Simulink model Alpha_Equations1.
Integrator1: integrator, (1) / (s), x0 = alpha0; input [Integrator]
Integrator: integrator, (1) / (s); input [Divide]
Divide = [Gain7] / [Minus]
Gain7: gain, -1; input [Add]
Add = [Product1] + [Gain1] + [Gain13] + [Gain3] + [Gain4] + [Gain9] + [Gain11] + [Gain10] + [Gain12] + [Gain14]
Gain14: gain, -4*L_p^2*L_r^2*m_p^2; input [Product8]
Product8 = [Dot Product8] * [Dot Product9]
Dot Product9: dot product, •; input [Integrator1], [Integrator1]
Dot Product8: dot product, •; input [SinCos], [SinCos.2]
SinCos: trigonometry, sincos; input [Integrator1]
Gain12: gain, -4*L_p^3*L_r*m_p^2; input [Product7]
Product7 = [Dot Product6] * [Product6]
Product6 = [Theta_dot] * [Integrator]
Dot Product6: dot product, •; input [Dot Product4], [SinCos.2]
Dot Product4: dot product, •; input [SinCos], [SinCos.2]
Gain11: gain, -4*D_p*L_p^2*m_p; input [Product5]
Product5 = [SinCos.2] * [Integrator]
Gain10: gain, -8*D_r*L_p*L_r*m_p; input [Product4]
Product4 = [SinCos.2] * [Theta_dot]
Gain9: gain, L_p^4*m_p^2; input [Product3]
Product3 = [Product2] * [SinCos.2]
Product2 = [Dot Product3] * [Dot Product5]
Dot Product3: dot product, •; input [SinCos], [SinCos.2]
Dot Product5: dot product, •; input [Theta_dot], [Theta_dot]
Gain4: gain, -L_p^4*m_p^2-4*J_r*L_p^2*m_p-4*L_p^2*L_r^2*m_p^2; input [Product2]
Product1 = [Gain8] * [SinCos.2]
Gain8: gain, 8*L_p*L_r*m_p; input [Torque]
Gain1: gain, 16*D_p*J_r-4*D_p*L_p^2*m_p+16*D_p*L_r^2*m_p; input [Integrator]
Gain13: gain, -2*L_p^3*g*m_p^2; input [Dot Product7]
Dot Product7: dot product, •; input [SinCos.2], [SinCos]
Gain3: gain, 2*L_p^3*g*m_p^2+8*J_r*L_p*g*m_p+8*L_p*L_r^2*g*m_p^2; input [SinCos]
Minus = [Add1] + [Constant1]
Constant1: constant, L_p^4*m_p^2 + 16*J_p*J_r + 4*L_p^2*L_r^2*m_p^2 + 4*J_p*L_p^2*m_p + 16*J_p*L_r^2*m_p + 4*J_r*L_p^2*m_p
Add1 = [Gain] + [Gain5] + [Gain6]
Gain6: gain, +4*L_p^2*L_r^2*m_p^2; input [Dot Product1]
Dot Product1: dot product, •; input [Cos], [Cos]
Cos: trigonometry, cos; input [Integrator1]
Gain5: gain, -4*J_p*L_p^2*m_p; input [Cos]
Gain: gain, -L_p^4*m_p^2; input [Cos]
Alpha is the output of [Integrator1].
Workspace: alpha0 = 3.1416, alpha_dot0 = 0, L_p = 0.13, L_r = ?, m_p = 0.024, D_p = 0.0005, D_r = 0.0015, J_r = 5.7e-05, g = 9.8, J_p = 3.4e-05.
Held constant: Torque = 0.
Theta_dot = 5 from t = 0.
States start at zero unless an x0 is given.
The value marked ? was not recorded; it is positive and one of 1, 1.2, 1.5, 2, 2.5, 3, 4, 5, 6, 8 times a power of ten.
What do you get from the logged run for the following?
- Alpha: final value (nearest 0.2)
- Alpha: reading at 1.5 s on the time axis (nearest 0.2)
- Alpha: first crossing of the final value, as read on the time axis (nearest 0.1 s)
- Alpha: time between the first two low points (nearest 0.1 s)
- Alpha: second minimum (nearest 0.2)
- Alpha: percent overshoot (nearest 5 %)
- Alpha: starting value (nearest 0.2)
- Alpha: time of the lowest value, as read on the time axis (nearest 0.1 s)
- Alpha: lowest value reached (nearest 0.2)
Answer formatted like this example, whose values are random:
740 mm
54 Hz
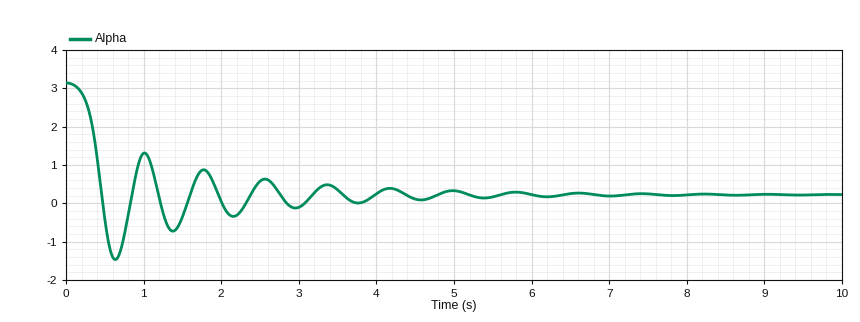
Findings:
0.2
-0.4
0.5 s
0.7 s
-0.8
60 %
3.2
0.6 s
-1.4
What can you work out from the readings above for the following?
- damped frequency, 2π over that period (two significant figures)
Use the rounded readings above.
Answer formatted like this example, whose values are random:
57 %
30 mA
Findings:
9.0 rad/s
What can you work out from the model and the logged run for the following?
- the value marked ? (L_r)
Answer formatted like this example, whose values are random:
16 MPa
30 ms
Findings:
0.15
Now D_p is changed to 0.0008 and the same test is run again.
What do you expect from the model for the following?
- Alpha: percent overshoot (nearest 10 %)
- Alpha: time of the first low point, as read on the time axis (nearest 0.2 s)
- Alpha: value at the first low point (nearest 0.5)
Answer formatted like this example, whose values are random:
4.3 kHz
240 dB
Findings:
50 %
0.6 s
-1.0
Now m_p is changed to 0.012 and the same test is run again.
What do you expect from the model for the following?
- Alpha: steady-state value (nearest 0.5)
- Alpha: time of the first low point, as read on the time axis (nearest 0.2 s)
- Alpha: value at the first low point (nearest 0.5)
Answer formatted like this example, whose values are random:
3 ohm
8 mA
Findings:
0.5
0.6 s
-1.0
